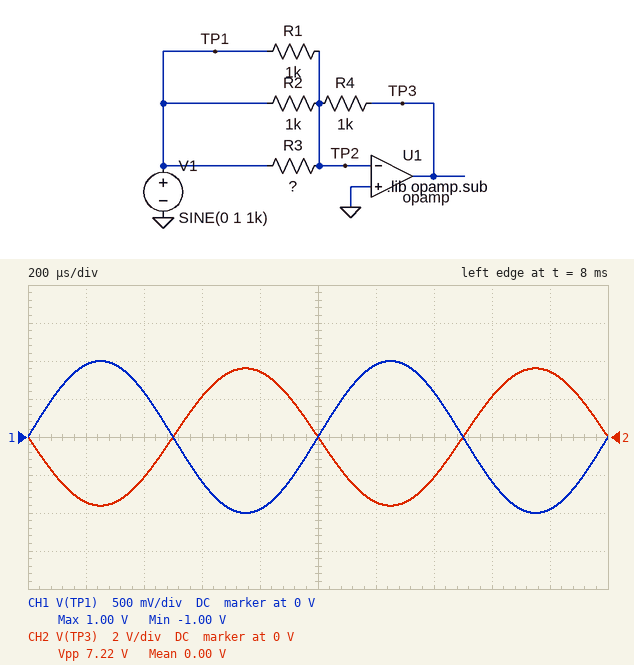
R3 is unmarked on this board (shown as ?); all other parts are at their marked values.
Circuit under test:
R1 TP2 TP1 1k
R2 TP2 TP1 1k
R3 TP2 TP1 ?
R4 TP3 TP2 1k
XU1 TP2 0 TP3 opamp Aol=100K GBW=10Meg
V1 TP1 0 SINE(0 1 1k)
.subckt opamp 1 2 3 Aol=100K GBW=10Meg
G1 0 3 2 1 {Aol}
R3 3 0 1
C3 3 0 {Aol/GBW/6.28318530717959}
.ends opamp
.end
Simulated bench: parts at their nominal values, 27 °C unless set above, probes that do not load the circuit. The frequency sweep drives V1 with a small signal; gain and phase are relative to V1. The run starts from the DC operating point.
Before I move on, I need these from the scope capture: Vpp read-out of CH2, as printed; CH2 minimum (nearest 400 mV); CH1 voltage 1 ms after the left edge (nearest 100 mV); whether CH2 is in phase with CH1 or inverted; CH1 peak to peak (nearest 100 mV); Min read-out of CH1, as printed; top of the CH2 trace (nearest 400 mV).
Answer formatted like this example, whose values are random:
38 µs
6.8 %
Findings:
7.22 V
-3.6 V
0 V
inverted
2.0 V
-1.00 V
3.6 V
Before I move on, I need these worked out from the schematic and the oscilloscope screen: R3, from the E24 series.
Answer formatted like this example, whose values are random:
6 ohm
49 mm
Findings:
620 Ω
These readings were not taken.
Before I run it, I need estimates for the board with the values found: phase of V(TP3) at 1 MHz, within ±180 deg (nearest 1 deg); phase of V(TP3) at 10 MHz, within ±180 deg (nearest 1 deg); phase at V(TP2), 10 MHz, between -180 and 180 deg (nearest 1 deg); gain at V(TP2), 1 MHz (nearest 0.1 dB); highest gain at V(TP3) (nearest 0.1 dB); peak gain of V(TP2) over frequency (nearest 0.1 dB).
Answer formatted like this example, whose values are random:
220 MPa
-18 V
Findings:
155 deg
102 deg
12 deg
-9.7 dB
11.2 dB
-2.1 dB
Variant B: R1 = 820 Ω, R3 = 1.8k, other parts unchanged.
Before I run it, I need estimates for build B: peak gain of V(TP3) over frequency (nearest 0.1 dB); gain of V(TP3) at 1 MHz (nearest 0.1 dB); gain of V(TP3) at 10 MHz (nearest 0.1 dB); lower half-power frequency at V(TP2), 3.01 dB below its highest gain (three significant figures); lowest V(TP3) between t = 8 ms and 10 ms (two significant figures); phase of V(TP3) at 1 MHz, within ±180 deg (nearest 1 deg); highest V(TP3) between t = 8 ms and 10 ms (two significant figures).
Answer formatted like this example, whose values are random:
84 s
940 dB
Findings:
8.9 dB
8.3 dB
-3.0 dB
2.65 MHz
-2.8 V
159 deg
2.8 V
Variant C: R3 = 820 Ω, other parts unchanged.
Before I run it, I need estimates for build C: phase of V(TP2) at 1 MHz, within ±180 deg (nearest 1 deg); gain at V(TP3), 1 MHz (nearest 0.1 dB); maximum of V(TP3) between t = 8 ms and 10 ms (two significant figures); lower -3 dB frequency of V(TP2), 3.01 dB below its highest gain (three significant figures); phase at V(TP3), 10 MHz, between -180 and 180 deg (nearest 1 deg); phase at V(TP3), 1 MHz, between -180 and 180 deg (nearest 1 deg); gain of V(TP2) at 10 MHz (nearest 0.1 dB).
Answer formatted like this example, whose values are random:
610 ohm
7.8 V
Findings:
67 deg
9.4 dB
3.2 V
2.37 MHz
103 deg
157 deg
-2.6 dB
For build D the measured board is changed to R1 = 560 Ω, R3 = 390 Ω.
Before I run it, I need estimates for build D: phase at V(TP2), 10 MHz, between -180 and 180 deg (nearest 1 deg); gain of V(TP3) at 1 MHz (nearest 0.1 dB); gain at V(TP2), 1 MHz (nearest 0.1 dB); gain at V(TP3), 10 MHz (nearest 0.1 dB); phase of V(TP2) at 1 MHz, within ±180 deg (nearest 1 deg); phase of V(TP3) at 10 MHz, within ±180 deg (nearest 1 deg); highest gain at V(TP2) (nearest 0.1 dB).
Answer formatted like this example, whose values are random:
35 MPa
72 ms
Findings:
9 deg
13.1 dB
-6.9 dB
-1.6 dB
58 deg
99 deg
-1.5 dB
